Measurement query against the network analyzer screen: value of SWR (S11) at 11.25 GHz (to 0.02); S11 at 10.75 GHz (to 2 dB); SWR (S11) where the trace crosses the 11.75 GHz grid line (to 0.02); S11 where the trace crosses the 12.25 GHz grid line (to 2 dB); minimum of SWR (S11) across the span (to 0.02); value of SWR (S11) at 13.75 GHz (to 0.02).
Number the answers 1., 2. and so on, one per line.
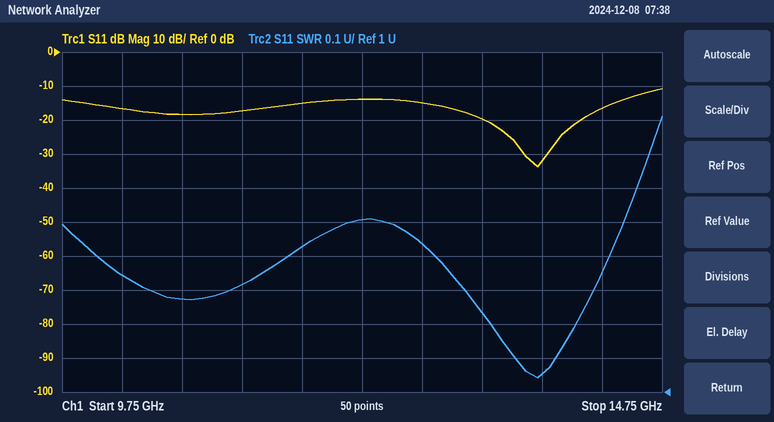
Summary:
1. 1.32
2. -18 dB
3. 1.42
4. -14 dB
5. 1.04
6. 1.06
